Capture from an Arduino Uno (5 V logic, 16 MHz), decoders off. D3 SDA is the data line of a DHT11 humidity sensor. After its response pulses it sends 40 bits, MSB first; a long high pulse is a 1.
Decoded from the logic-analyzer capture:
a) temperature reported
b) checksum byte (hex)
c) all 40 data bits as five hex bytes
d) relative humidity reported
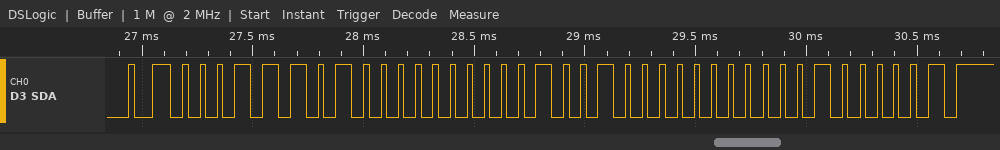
36.0 °C
0x41
1D 00 24 00 41
29 %
